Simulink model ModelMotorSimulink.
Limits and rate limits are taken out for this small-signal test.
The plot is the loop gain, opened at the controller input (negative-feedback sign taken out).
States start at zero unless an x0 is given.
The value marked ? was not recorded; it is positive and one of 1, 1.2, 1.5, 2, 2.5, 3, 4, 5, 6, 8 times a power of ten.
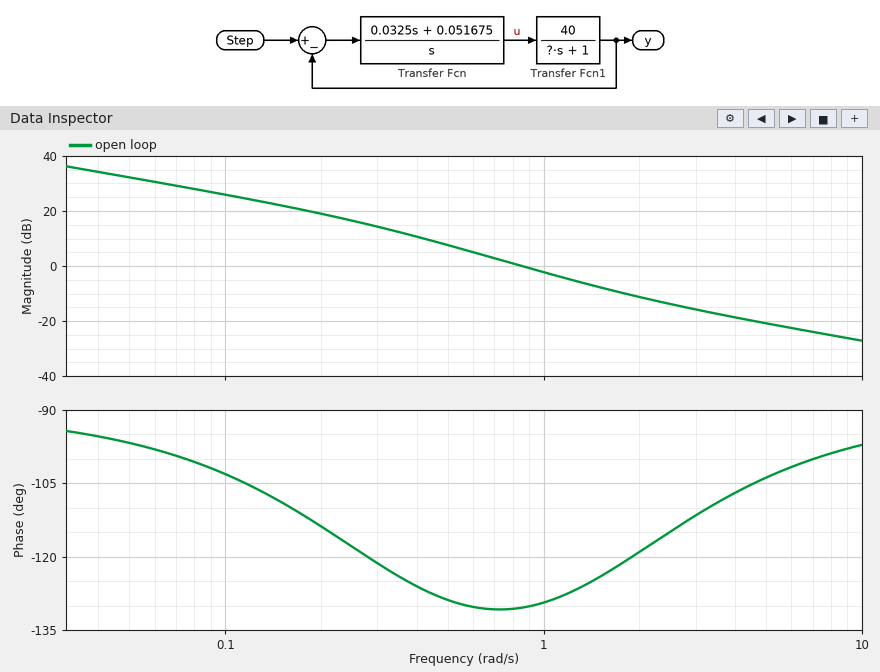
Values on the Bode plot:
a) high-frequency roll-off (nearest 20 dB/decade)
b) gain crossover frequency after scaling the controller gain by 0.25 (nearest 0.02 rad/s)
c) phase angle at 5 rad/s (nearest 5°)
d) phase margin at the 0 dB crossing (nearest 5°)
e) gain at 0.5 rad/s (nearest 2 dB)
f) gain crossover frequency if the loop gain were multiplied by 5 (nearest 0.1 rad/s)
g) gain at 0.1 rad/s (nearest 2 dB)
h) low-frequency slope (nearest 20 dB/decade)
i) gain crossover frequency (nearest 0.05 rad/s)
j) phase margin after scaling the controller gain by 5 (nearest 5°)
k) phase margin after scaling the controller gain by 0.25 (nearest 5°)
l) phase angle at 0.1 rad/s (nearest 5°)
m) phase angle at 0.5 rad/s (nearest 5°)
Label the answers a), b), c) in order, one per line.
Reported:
a) -20 dB/decade
b) 0.36 rad/s
c) -105°
d) 50°
e) 8 dB
f) 2.5 rad/s
g) 26 dB
h) -20 dB/decade
i) 0.85 rad/s
j) 65°
k) 55°
l) -105°
m) -130°
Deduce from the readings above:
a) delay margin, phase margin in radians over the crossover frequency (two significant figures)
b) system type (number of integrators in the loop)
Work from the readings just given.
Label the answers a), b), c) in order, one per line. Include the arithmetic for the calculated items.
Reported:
a) 50 × π / 180 / 0.85 = 1.0 s
b) 1
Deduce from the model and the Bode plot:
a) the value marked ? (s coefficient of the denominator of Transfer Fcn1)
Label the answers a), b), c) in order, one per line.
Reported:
a) 3
